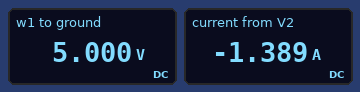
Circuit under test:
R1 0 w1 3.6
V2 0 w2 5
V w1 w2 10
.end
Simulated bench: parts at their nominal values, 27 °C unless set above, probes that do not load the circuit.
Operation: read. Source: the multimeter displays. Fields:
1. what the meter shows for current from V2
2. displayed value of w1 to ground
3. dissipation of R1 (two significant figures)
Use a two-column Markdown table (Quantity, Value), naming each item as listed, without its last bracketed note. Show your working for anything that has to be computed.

| Quantity | Value |
|---|---|
| what the meter shows for current from V2 | -1.389 A |
| displayed value of w1 to ground | 5.000 V |
| dissipation of R1 | (5 V)^2 / 3.6 Ω = 6.9 W |
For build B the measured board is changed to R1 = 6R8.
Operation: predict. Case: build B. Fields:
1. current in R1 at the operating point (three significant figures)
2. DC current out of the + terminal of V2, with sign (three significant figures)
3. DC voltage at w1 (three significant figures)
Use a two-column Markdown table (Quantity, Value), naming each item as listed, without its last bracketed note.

| Quantity | Value |
|---|---|
| current in R1 at the operating point | 735 mA |
| DC current out of the + terminal of V2, with sign | -735 mA |
| DC voltage at w1 | 5.00 V |
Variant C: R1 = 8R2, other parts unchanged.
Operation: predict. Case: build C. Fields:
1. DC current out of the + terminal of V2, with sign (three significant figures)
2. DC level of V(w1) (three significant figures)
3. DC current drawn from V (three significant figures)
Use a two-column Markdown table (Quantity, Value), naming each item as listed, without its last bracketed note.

| Quantity | Value |
|---|---|
| DC current out of the + terminal of V2, with sign | -610 mA |
| DC level of V(w1) | 5.00 V |
| DC current drawn from V | 610 mA |
